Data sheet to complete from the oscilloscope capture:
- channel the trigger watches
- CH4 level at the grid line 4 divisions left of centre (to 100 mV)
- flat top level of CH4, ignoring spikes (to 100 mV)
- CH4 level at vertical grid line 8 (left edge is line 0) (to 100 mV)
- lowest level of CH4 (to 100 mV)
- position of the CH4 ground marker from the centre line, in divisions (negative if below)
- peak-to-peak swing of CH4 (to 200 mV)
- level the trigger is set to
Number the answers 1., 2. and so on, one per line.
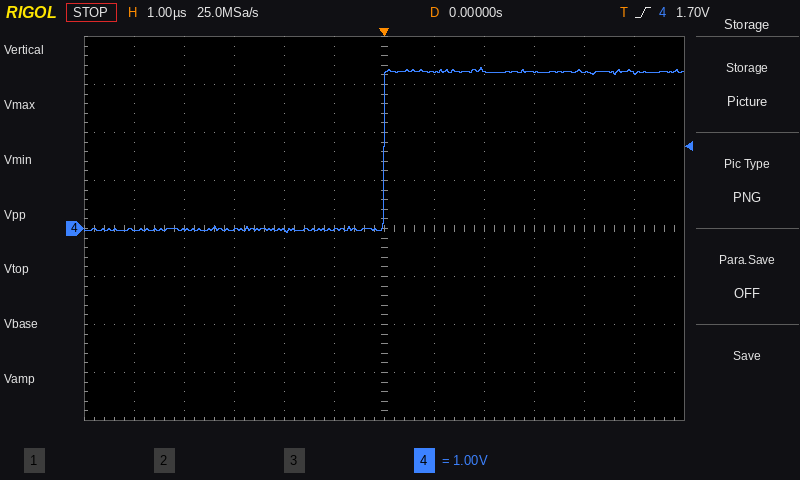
1. CH4
2. 0.0 V
3. 3.3 V
4. 3.3 V
5. -100 mV
6. 0.0 div
7. 3.4 V
8. 1.70 V
